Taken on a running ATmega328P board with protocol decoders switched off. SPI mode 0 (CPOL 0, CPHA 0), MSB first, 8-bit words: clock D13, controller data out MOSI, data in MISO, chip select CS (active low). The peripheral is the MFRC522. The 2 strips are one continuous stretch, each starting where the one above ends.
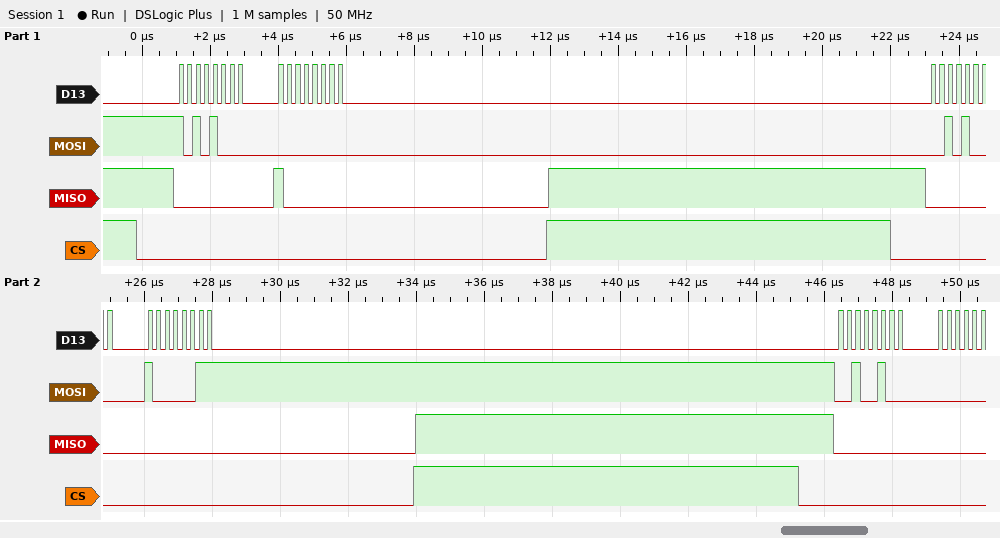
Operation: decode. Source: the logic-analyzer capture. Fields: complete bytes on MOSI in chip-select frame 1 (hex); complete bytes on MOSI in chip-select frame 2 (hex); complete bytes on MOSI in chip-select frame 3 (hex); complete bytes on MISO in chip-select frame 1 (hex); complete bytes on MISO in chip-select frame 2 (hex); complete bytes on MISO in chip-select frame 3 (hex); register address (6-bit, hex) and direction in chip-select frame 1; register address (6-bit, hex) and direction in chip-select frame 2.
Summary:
A8 00
28 83
24
00 80
00 00
00
0x14 read
0x14 write
